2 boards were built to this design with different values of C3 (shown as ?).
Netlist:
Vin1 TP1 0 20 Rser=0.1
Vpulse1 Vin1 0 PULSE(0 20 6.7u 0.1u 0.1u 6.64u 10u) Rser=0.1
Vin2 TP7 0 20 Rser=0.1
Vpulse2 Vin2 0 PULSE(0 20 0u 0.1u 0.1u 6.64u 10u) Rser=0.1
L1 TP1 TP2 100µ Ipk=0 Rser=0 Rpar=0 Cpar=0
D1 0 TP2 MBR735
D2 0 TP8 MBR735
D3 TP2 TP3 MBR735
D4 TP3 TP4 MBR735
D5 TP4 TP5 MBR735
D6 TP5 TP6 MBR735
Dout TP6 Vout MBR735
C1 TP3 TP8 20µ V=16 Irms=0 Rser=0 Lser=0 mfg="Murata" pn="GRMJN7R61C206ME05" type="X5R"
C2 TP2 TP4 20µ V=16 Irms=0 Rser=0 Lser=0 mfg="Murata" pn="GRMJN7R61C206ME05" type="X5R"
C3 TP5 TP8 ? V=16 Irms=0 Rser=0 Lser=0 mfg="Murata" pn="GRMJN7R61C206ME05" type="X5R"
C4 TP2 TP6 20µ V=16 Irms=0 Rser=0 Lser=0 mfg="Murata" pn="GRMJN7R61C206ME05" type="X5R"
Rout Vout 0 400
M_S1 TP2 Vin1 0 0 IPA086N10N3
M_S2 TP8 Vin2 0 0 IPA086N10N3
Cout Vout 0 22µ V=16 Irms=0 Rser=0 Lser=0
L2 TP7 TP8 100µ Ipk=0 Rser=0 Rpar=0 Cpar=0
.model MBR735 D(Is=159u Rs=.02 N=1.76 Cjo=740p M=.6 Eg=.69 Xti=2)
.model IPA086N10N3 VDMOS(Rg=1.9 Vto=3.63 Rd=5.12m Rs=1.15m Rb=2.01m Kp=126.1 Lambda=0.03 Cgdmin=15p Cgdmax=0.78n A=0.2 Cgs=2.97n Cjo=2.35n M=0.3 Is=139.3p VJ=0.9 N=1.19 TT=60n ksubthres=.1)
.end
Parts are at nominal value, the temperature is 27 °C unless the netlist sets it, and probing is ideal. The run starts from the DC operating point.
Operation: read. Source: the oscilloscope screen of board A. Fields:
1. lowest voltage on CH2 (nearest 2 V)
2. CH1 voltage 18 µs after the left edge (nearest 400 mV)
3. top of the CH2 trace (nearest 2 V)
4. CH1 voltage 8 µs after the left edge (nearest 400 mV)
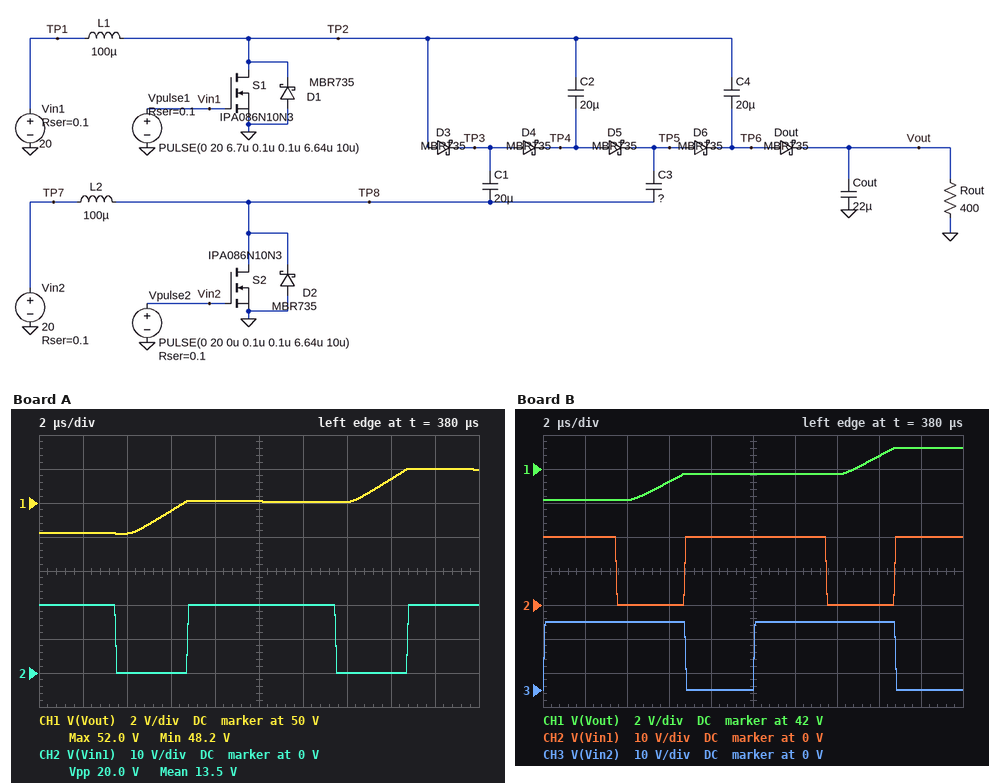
0 V
52.0 V
20 V
50.0 V
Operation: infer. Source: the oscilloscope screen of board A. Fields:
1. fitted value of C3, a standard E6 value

6.8 µF
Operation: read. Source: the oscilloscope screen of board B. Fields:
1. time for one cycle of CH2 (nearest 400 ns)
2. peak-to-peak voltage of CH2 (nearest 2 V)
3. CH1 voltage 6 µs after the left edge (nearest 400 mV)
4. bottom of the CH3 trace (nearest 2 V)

10.0 µs
20 V
41.2 V
0 V
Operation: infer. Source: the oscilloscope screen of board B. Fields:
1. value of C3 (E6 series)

47 µF
